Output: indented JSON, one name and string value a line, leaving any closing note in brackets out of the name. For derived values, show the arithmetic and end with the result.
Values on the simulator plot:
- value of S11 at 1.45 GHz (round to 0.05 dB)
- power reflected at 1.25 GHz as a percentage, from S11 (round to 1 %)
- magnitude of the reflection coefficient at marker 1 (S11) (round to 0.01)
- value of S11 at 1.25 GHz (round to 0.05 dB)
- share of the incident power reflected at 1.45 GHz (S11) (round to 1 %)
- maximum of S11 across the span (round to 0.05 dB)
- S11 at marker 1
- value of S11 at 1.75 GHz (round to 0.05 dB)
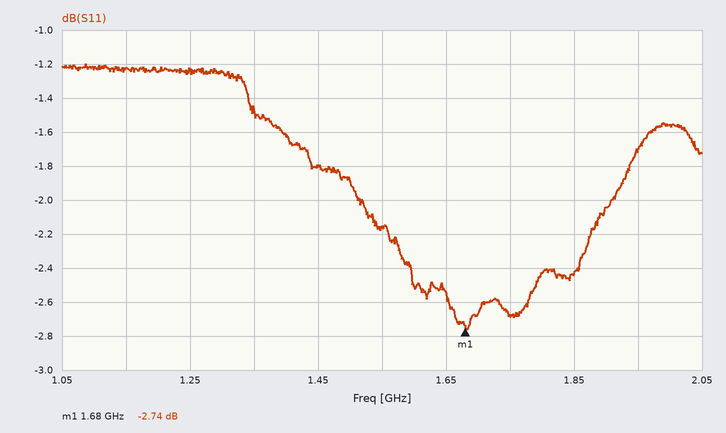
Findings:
{
  "value of S11 at 1.45 GHz": "-1.80 dB",
  "power reflected at 1.25 GHz as a percentage, from S11": "10^(-1.25/10) ≈ 75 %",
  "magnitude of the reflection coefficient at marker 1 (S11)": "10^(-2.74/20) ≈ 0.73",
  "value of S11 at 1.25 GHz": "-1.25 dB",
  "share of the incident power reflected at 1.45 GHz (S11)": "10^(-1.8/10) ≈ 66 %",
  "maximum of S11 across the span": "-1.20 dB",
  "S11 at marker 1": "-2.74 dB",
  "value of S11 at 1.75 GHz": "-2.70 dB"
}
